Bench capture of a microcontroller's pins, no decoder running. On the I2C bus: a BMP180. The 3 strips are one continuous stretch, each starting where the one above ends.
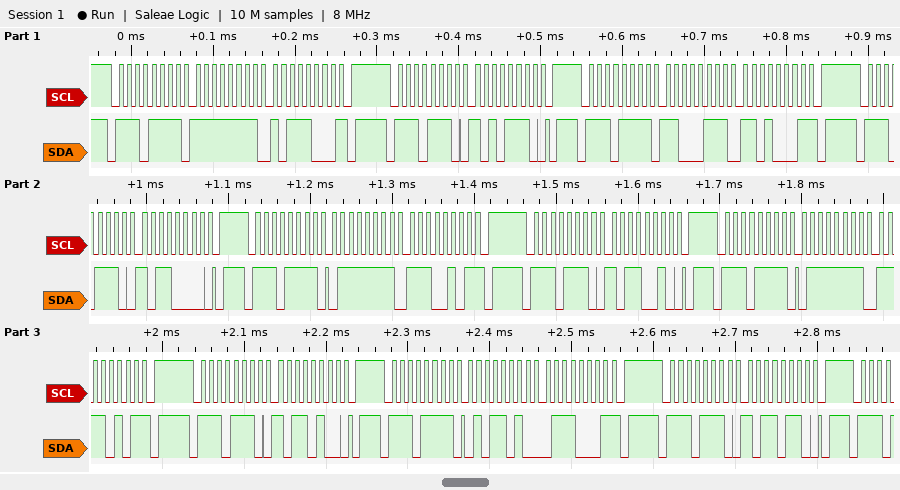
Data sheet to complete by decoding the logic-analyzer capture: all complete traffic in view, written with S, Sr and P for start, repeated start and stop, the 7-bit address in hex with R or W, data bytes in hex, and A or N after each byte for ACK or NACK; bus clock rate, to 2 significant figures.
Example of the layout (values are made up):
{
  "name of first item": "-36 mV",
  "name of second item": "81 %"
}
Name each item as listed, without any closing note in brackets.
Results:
{
  "all complete traffic in view, written with S, Sr and P for start, repeated start and stop, the 7-bit address in hex with R or W, data bytes in hex, and A or N after each byte for ACK or NACK": "S 77R A FF A B8 N P S 77W A AE A P S 77R A C7 A D1 N P S 77W A B0 A P S 77R A 7F A E5 N P S 77W A B2 A P S 77R A 7F A F5 N P S 77W A B4 A P S 77R A 5A A 71 N P S 77W A B6 A P",
  "bus clock rate, to 2 significant figures": "100 kHz"
}
